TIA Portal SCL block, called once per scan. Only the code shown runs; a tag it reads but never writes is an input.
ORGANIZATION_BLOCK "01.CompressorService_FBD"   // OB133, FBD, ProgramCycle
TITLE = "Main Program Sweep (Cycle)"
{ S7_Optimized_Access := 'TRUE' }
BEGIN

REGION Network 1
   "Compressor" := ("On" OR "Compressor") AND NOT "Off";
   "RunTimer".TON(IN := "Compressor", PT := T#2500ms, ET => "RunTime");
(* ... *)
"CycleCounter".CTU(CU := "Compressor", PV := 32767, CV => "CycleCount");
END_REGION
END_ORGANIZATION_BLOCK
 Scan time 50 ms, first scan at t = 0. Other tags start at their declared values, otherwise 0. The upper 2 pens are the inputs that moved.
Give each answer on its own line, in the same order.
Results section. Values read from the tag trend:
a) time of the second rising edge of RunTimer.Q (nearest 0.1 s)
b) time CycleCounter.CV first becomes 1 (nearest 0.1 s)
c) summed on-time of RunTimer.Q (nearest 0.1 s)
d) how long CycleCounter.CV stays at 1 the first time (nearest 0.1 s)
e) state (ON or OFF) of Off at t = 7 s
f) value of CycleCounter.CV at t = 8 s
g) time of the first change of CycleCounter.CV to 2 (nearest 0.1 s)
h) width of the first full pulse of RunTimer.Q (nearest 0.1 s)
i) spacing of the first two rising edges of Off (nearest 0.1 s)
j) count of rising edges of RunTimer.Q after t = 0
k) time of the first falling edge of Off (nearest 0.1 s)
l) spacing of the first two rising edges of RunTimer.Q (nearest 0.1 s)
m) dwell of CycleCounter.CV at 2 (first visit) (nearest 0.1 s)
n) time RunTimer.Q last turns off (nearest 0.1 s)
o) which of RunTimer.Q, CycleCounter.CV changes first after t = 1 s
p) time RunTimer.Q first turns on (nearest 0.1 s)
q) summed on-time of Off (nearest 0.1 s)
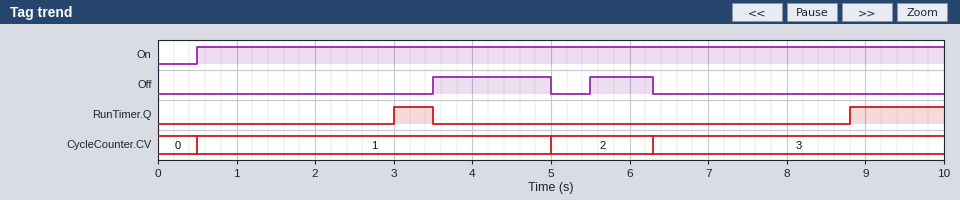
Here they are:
8.8 s
0.5 s
1.7 s
4.5 s
OFF
3
5.0 s
0.5 s
2.0 s
2
5.0 s
5.8 s
1.3 s
3.5 s
RunTimer.Q
3.0 s
2.3 s
